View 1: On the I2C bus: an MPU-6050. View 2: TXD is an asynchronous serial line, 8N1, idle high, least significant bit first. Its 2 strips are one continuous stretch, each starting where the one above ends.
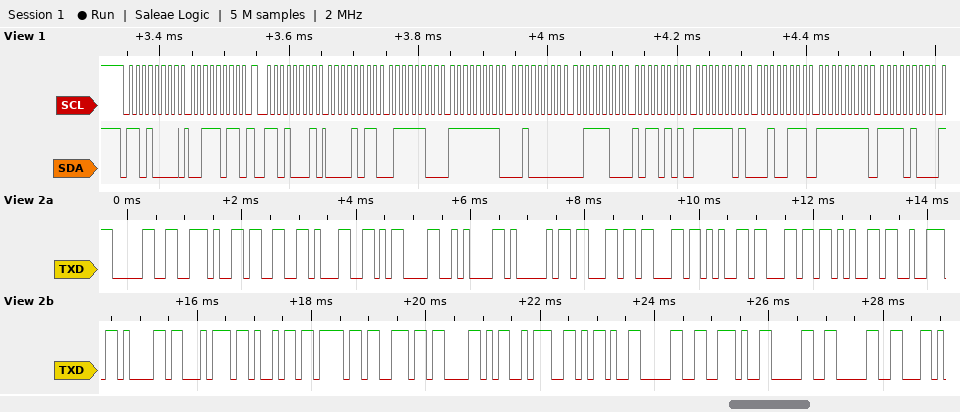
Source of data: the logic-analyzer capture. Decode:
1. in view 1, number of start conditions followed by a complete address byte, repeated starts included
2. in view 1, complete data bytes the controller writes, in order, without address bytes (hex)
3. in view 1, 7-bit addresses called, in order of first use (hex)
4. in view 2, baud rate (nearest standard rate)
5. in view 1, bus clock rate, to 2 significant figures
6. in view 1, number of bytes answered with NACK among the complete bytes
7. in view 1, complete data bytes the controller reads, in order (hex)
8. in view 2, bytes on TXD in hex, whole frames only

2
3B
0x68
9600 baud
100 kHz
0
0B 7C FF 20 3C B5 FD 27 FF F4
30 2E 33 31 0D 0A 41 63 63 65 6C 65 72 61 74 69 6F 6E 58 3A 2D 30 2E 30 30
